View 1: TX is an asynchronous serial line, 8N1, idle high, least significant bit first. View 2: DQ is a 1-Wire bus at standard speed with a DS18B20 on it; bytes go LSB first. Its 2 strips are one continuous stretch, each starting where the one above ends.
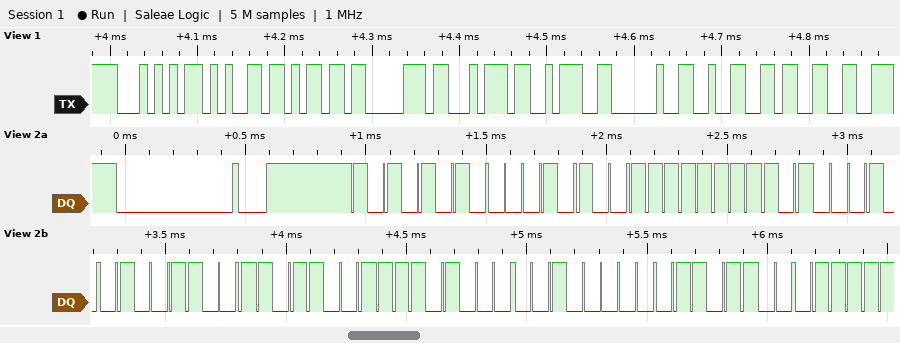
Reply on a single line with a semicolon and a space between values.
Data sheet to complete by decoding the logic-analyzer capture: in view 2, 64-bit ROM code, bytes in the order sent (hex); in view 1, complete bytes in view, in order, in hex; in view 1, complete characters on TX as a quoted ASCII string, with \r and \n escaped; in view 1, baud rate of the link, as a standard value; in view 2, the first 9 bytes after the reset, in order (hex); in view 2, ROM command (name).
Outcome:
28 FF 45 32 9B 17 04 36; 54 65 6D 70 74 3A 20 32 33; "Tempt: 23"; 115200 baud; 55 28 FF 45 32 9B 17 04 36; Match ROM
